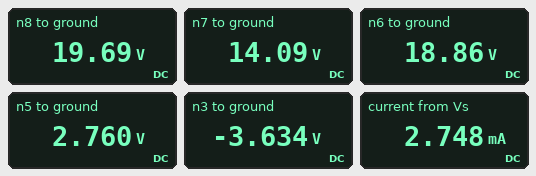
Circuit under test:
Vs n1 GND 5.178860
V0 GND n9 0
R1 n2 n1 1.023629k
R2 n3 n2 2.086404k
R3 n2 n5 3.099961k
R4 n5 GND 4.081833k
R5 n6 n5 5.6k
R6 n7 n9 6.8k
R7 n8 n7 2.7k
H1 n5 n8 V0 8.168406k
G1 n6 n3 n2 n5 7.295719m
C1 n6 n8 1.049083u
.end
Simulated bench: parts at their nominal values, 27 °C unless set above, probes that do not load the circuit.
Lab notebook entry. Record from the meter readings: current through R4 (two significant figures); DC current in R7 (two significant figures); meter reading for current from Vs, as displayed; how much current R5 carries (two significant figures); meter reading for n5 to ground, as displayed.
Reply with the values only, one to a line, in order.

680 µA
2.1 mA
2.748 mA
2.9 mA
2.760 V
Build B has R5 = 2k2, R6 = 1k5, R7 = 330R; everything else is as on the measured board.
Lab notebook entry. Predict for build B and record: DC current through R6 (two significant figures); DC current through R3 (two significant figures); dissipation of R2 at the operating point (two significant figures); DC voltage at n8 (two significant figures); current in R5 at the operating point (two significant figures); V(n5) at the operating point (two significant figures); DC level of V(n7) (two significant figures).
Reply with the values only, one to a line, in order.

760 µA
19 µA
400 µW
-1.4 V
440 µA
4.8 V
-1.1 V
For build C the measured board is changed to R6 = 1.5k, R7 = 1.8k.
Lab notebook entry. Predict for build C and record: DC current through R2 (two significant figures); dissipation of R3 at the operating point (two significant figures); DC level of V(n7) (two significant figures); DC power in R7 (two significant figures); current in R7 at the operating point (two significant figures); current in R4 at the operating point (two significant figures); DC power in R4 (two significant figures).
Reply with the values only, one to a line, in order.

210 µA
260 nW
-1.5 V
1.9 mW
1.0 mA
1.2 mA
6.1 mW
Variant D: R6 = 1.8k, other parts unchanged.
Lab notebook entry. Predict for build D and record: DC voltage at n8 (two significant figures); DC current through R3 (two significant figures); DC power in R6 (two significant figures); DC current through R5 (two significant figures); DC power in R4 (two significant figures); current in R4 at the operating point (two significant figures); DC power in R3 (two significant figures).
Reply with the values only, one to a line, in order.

-6.5 V
6.8 µA
3.8 mW
150 µA
6.9 mW
1.3 mA
140 nW
